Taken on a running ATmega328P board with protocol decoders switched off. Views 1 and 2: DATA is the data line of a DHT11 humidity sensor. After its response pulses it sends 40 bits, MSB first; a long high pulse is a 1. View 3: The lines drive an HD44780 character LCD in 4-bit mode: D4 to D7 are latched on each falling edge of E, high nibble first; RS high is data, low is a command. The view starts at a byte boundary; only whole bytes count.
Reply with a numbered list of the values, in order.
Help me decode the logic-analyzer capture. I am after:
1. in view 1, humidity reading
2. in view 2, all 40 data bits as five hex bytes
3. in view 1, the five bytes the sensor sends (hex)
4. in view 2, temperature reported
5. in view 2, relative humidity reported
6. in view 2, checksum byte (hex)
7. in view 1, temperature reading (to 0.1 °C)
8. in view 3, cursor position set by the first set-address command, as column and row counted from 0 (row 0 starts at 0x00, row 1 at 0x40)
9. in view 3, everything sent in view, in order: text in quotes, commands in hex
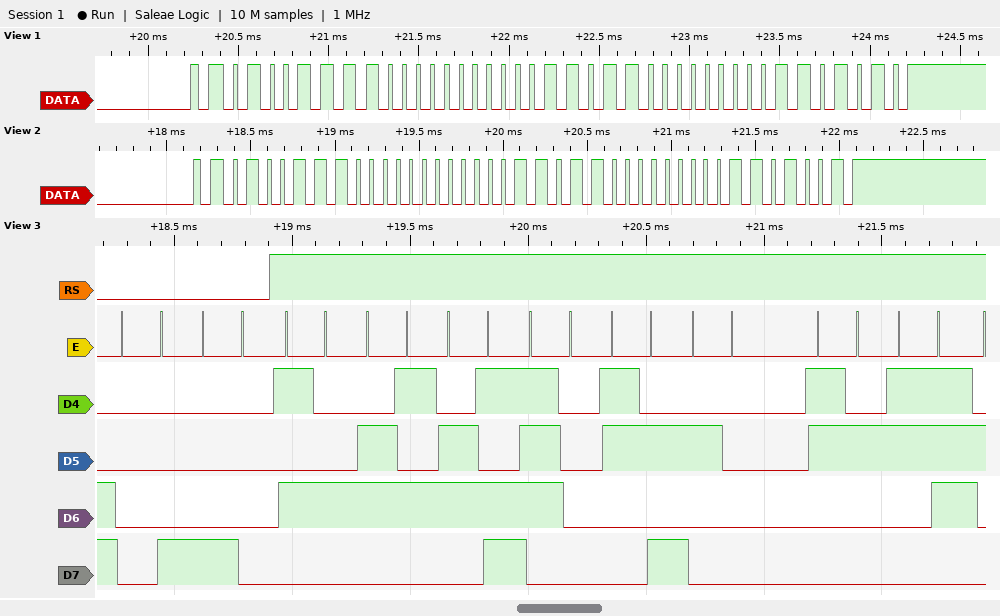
1. 79 %
2. 4E 00 1B 00 69
3. 4F 00 1B 00 6A
4. 27.0 °C
5. 78 %
6. 0x69
7. 27.0 °C
8. column 0, row 0
9. 0x08 0x80 "Temp: 27"
